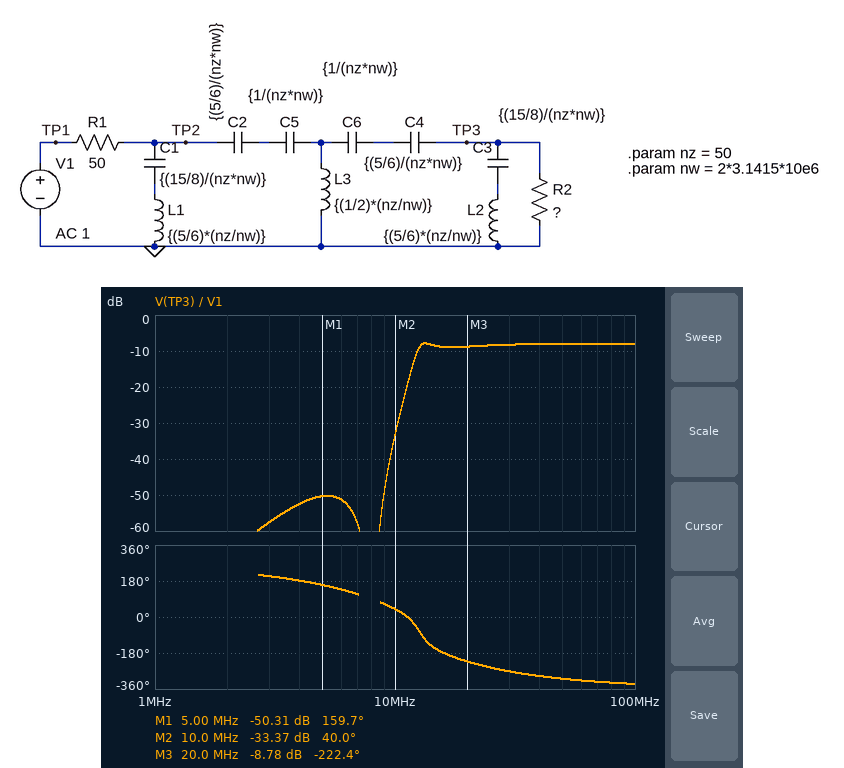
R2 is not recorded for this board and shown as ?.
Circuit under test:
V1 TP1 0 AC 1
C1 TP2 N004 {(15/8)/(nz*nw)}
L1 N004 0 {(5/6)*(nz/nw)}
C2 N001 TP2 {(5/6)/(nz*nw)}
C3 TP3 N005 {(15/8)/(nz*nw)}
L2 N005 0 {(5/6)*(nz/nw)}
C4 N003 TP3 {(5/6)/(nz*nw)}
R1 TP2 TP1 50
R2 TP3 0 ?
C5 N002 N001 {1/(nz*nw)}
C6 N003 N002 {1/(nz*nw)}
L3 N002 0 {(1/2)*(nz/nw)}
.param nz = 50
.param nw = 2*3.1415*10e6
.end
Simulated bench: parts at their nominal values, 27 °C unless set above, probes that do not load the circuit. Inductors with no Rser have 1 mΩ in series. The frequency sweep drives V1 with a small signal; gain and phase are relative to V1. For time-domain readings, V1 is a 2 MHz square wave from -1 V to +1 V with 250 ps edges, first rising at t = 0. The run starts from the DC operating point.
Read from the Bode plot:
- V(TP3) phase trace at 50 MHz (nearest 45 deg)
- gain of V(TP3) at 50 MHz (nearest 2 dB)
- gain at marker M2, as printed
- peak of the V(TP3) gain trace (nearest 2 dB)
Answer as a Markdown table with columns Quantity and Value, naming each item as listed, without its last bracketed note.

| Quantity | Value |
|---|---|
| V(TP3) phase trace at 50 MHz | -315 deg |
| gain of V(TP3) at 50 MHz | -8 dB |
| gain at marker M2, as printed | -33.37 dB |
| peak of the V(TP3) gain trace | -8 dB |
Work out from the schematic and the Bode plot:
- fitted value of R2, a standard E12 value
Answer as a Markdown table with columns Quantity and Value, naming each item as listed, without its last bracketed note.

| Quantity | Value |
|---|---|
| fitted value of R2, a standard E12 value | 33 Ω |
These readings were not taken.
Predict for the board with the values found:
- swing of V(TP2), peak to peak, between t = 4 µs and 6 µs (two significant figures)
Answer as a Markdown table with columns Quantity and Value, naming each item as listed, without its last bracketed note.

| Quantity | Value |
|---|---|
| swing of V(TP2), peak to peak, between t = 4 µs and 6 µs | 2.1 V |
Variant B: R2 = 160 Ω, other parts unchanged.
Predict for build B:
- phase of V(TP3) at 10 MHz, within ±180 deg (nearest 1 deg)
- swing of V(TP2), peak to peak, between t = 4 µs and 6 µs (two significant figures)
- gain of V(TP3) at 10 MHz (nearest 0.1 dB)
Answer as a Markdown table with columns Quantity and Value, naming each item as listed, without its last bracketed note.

| Quantity | Value |
|---|---|
| phase of V(TP3) at 10 MHz, within ±180 deg | 63 deg |
| swing of V(TP2), peak to peak, between t = 4 µs and 6 µs | 2.1 V |
| gain of V(TP3) at 10 MHz | -32.2 dB |
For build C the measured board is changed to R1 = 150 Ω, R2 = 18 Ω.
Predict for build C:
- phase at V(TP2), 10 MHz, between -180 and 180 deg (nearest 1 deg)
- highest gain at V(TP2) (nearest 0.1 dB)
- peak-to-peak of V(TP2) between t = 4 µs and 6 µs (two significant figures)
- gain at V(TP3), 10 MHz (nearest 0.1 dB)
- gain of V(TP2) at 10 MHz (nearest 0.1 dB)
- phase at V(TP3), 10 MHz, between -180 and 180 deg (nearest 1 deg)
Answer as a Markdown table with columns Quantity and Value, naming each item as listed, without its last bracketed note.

| Quantity | Value |
|---|---|
| phase at V(TP2), 10 MHz, between -180 and 180 deg | 83 deg |
| highest gain at V(TP2) | 0 dB |
| peak-to-peak of V(TP2) between t = 4 µs and 6 µs | 1.7 V |
| gain at V(TP3), 10 MHz | -44.4 dB |
| gain of V(TP2) at 10 MHz | -18.2 dB |
| phase at V(TP3), 10 MHz, between -180 and 180 deg | 37 deg |
